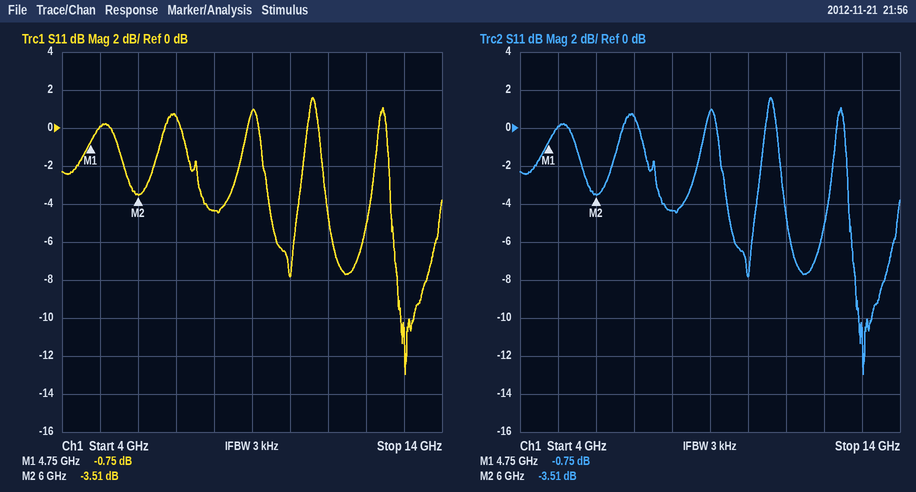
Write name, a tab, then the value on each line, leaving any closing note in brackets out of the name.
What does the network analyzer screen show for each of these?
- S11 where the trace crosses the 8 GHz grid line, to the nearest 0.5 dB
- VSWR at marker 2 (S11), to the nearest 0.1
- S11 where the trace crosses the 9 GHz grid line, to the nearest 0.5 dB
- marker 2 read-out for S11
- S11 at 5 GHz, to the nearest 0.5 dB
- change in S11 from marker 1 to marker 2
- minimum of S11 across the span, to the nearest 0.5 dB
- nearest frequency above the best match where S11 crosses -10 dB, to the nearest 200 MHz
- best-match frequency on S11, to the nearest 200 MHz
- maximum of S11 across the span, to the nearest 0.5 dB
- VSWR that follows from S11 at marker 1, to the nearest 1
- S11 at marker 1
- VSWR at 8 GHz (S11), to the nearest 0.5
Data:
S11 where the trace crosses the 8 GHz grid line, to the nearest 0.5 dB	-4.5 dB
VSWR at marker 2 (S11), to the nearest 0.1	5.0
S11 where the trace crosses the 9 GHz grid line, to the nearest 0.5 dB	1.0 dB
marker 2 read-out for S11	-3.51 dB
S11 at 5 GHz, to the nearest 0.5 dB	0.0 dB
change in S11 from marker 1 to marker 2	-2.76 dB
minimum of S11 across the span, to the nearest 0.5 dB	-13.0 dB
nearest frequency above the best match where S11 crosses -10 dB, to the nearest 200 MHz	13.2 GHz
best-match frequency on S11, to the nearest 200 MHz	13.0 GHz
maximum of S11 across the span, to the nearest 0.5 dB	1.5 dB
VSWR that follows from S11 at marker 1, to the nearest 1	23
S11 at marker 1	-0.75 dB
VSWR at 8 GHz (S11), to the nearest 0.5	4.0
